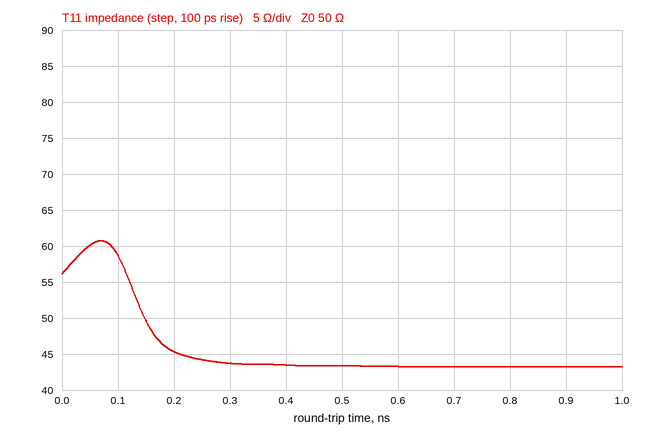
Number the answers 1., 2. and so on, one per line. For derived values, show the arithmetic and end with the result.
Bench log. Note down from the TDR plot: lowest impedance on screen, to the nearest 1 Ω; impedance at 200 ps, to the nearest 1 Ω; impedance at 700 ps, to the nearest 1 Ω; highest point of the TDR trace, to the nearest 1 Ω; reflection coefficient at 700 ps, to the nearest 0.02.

1. 43 Ω
2. 45 Ω
3. 43 Ω
4. 61 Ω
5. (43 − 50)/(43 + 50) ≈ -0.08
